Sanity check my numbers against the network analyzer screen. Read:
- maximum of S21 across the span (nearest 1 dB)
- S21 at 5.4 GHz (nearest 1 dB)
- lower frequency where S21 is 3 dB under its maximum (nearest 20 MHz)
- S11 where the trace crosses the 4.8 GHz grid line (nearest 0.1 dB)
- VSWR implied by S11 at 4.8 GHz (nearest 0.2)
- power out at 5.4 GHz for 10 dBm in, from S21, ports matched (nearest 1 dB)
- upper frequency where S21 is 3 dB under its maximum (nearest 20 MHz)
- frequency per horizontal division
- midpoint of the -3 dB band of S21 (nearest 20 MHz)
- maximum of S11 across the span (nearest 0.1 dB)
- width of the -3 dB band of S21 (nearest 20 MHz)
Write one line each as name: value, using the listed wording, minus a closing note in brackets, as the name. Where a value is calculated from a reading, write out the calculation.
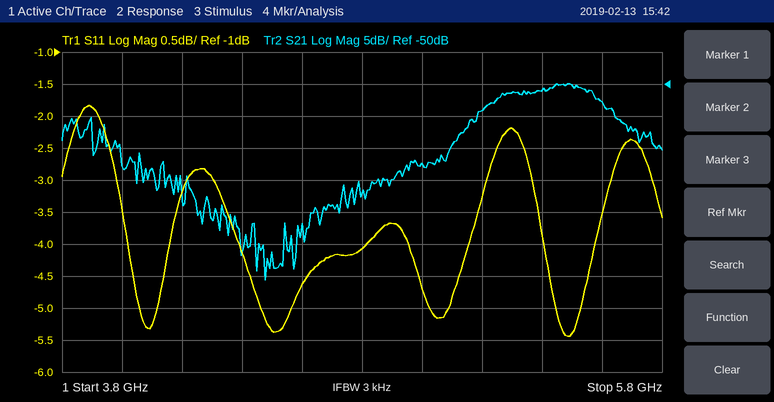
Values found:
maximum of S21 across the span: -50 dB
S21 at 5.4 GHz: -51 dB
lower frequency where S21 is 3 dB under its maximum: 5.24 GHz
S11 where the trace crosses the 4.8 GHz grid line: -4.1 dB
VSWR implied by S11 at 4.8 GHz: |Γ| = 10^(-4.1/20) = 0.6237; VSWR = (1 + 0.6237)/(1 − 0.6237) ≈ 4.32, so 4.4 to the nearest 0.2
power out at 5.4 GHz for 10 dBm in, from S21, ports matched: 10 dBm + (-51 dB) = -41 dBm
upper frequency where S21 is 3 dB under its maximum: 5.60 GHz
frequency per horizontal division: 200 MHz
midpoint of the -3 dB band of S21: 5.42 GHz
maximum of S11 across the span: -1.8 dB
width of the -3 dB band of S21: 5.60 GHz − 5.24 GHz = 360 MHz
